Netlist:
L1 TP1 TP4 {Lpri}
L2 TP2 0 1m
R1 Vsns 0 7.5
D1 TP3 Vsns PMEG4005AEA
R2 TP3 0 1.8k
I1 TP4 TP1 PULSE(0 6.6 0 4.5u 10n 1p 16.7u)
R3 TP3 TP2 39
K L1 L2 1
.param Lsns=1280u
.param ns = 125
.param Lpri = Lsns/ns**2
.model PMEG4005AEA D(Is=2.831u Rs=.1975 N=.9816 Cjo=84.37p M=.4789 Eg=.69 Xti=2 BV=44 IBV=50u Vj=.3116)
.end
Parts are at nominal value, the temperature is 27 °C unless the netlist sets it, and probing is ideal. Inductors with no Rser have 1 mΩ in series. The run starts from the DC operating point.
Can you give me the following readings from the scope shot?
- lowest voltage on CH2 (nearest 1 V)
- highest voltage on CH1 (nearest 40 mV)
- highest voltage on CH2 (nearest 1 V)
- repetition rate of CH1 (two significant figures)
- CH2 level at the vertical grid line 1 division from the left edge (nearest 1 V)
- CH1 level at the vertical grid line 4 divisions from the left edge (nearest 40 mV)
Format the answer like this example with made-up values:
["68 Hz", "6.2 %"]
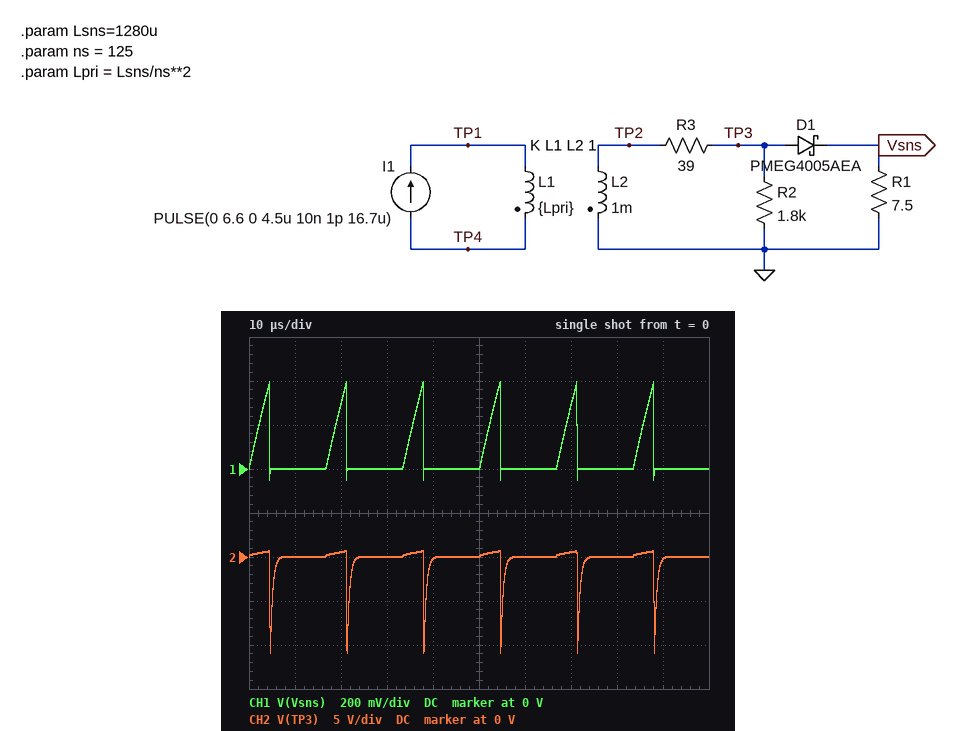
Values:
["-11 V", "400 mV", "1 V", "60 kHz", "0 V", "0 V"]
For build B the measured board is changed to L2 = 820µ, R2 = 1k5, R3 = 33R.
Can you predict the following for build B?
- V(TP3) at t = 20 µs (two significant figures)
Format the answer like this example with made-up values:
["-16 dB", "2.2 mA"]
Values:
["580 mV"]
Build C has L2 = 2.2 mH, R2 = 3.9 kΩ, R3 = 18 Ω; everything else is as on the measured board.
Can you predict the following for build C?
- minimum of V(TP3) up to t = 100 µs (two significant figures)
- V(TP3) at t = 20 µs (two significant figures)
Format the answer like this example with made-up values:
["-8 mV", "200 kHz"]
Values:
["-4.4 V", "450 mV"]
